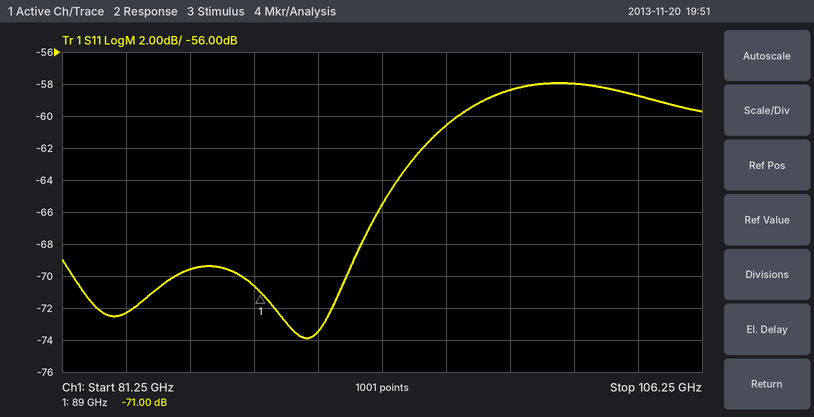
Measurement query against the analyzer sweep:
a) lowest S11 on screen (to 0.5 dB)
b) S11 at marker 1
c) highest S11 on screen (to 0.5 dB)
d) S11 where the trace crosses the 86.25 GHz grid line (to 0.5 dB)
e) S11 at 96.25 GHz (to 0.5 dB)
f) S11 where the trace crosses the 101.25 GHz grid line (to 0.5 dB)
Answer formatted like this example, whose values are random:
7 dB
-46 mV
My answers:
-74.0 dB
-71.00 dB
-58.0 dB
-69.5 dB
-60.5 dB
-58.0 dB
